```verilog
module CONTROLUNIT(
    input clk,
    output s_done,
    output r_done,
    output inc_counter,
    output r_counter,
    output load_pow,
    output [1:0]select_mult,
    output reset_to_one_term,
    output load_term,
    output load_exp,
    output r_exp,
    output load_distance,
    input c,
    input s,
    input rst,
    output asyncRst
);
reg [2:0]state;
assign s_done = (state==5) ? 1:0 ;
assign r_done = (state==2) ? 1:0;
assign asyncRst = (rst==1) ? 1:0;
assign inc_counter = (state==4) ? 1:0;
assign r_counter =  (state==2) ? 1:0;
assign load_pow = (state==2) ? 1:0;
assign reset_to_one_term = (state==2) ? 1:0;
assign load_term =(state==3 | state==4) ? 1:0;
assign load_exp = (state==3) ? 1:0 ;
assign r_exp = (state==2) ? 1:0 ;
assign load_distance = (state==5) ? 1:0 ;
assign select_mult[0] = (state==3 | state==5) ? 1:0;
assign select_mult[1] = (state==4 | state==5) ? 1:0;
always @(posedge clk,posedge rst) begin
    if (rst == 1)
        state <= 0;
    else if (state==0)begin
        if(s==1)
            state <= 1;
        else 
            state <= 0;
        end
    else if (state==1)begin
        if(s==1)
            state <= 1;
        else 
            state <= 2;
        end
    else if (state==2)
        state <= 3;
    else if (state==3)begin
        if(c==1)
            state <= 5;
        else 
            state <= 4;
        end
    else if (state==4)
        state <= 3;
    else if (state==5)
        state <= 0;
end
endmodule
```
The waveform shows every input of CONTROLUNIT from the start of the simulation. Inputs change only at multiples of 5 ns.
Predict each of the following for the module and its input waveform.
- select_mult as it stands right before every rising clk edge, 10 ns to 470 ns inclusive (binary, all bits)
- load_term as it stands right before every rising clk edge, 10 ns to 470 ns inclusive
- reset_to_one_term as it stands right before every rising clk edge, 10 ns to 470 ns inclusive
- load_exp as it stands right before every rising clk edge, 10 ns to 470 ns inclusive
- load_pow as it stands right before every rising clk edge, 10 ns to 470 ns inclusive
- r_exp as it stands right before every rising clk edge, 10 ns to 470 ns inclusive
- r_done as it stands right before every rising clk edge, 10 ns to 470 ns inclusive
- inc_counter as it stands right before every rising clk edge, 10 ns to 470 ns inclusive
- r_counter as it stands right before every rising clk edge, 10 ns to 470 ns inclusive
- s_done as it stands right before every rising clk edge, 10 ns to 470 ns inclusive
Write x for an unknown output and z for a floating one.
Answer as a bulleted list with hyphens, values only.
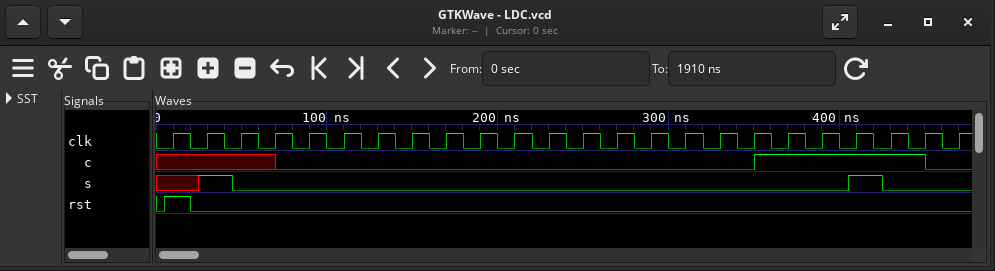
- 00, 00, 00, 00, 01, 10, 01, 10, 01, 10, 01, 10, 01, 10, 01, 10, 01, 10, 01, 11, 00, 00, 00, 01
- 0 0 0 0 1 1 1 1 1 1 1 1 1 1 1 1 1 1 1 0 0 0 0 1
- 0 0 0 1 0 0 0 0 0 0 0 0 0 0 0 0 0 0 0 0 0 0 1 0
- 0 0 0 0 1 0 1 0 1 0 1 0 1 0 1 0 1 0 1 0 0 0 0 1
- 0 0 0 1 0 0 0 0 0 0 0 0 0 0 0 0 0 0 0 0 0 0 1 0
- 0 0 0 1 0 0 0 0 0 0 0 0 0 0 0 0 0 0 0 0 0 0 1 0
- 0 0 0 1 0 0 0 0 0 0 0 0 0 0 0 0 0 0 0 0 0 0 1 0
- 0 0 0 0 0 1 0 1 0 1 0 1 0 1 0 1 0 1 0 0 0 0 0 0
- 0 0 0 1 0 0 0 0 0 0 0 0 0 0 0 0 0 0 0 0 0 0 1 0
- 0 0 0 0 0 0 0 0 0 0 0 0 0 0 0 0 0 0 0 1 0 0 0 0
